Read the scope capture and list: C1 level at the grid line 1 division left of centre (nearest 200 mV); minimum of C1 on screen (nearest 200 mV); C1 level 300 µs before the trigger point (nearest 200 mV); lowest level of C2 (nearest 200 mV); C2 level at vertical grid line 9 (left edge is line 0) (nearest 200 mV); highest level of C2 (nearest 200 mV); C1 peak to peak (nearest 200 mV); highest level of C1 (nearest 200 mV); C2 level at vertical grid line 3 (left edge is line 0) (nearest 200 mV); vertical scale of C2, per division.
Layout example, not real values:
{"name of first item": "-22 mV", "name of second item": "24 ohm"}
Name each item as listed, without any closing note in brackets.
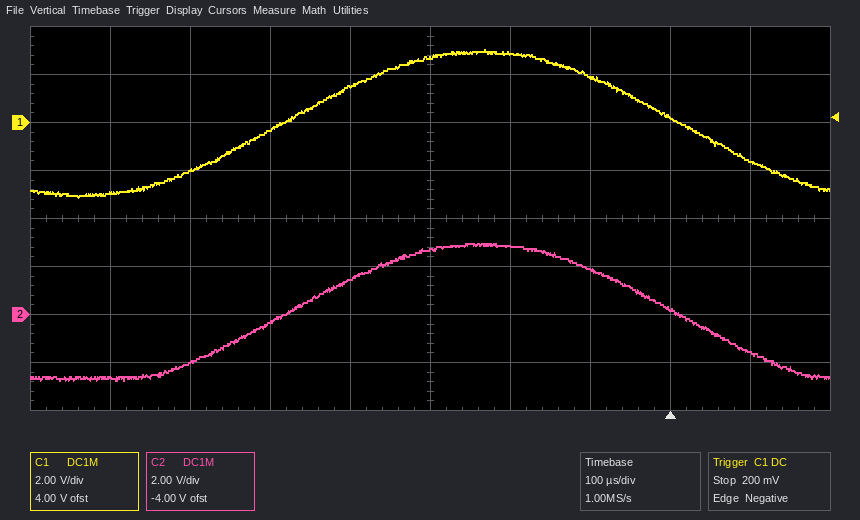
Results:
{"C1 level at the grid line 1 division left of centre": "1.6 V", "minimum of C1 on screen": "-3.2 V", "C1 level 300 µs before the trigger point": "2.8 V", "lowest level of C2": "-2.8 V", "C2 level at vertical grid line 9 (left edge is line 0)": "-1.6 V", "highest level of C2": "3.0 V", "C1 peak to peak": "6.2 V", "highest level of C1": "3.0 V", "C2 level at vertical grid line 3 (left edge is line 0)": "-400 mV", "vertical scale of C2, per division": "2 V"}
